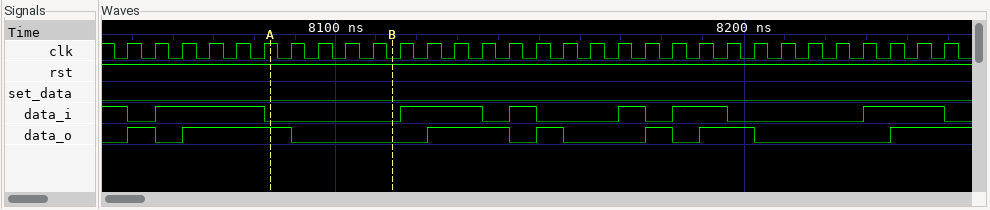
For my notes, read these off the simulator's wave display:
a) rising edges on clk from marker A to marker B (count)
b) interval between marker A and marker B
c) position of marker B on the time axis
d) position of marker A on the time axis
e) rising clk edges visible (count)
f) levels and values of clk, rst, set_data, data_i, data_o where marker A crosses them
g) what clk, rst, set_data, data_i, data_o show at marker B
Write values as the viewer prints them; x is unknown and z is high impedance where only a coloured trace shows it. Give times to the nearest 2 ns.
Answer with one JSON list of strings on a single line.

["4", "30 ns", "8114 ns", "8084 ns", "31", "clk=1, rst=1, set_data=0, data_i=0, data_o=1", "clk=0, rst=1, set_data=0, data_i=0, data_o=0"]
